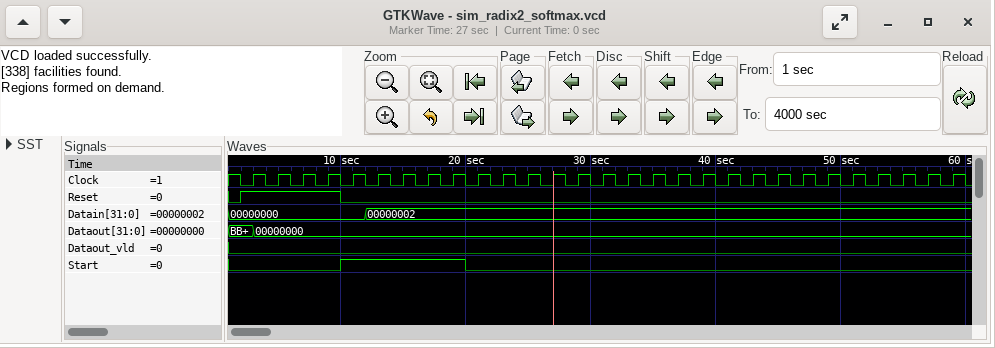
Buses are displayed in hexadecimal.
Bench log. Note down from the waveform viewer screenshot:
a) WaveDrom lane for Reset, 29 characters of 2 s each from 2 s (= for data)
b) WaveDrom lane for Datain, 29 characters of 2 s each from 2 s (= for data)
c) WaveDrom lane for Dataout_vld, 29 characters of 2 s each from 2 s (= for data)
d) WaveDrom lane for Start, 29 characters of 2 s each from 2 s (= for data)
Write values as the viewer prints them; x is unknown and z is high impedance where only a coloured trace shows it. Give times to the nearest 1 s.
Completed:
{name: 'Reset', wave: '1...0........................'}
{name: 'Datain', wave: '=....=.......................', data: '00000000 00000002'}
{name: 'Dataout_vld', wave: '0............................'}
{name: 'Start', wave: '0...1....0...................'}
